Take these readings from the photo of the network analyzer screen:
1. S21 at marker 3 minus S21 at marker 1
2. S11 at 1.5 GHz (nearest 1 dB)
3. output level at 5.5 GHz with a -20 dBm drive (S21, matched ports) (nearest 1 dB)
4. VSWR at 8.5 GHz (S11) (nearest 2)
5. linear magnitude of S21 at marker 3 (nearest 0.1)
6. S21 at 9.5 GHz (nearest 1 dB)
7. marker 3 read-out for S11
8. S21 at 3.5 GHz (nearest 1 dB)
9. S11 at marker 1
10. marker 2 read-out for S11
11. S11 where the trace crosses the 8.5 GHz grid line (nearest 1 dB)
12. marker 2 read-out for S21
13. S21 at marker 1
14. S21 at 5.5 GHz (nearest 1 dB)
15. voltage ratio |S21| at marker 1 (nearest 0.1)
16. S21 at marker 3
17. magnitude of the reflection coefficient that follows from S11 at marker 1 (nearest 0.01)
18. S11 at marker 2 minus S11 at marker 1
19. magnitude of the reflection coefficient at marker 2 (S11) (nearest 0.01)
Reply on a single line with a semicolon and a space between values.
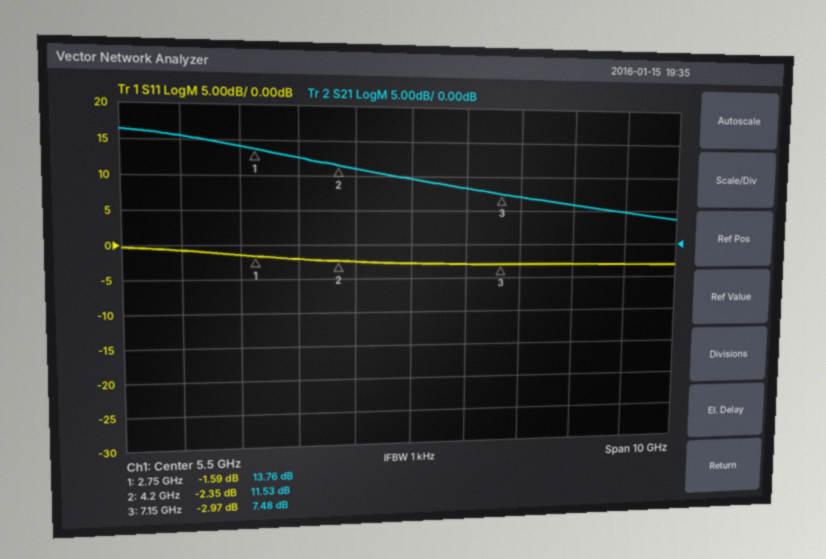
-6.28 dB; -1 dB; -10 dBm; 6; 2.4; 5 dB; -2.97 dB; 13 dB; -1.59 dB; -2.35 dB; -3 dB; 11.53 dB; 13.76 dB; 10 dB; 4.9; 7.48 dB; 0.83; -0.76 dB; 0.76
